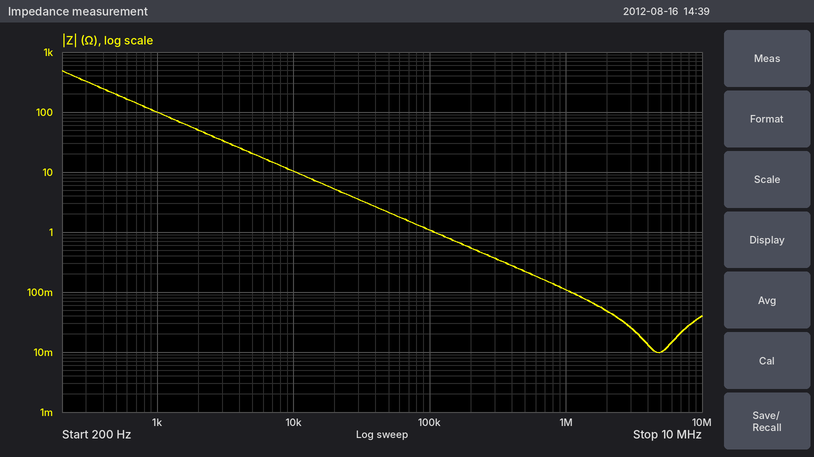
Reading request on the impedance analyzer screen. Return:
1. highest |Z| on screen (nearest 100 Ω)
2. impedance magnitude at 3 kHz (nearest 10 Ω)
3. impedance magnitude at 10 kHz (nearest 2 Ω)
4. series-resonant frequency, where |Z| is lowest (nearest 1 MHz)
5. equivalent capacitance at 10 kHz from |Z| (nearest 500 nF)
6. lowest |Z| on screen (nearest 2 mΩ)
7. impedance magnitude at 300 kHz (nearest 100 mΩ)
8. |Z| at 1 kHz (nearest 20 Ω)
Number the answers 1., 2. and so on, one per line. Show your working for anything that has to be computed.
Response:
1. 500 Ω
2. 30 Ω
3. 10 Ω
4. 5 MHz
5. C = 1/(2π × 10 kHz × 10 Ω) ≈ 1.59 µF, so 1.5 µF to the nearest 500 nF
6. 10 mΩ
7. 400 mΩ
8. 100 Ω
